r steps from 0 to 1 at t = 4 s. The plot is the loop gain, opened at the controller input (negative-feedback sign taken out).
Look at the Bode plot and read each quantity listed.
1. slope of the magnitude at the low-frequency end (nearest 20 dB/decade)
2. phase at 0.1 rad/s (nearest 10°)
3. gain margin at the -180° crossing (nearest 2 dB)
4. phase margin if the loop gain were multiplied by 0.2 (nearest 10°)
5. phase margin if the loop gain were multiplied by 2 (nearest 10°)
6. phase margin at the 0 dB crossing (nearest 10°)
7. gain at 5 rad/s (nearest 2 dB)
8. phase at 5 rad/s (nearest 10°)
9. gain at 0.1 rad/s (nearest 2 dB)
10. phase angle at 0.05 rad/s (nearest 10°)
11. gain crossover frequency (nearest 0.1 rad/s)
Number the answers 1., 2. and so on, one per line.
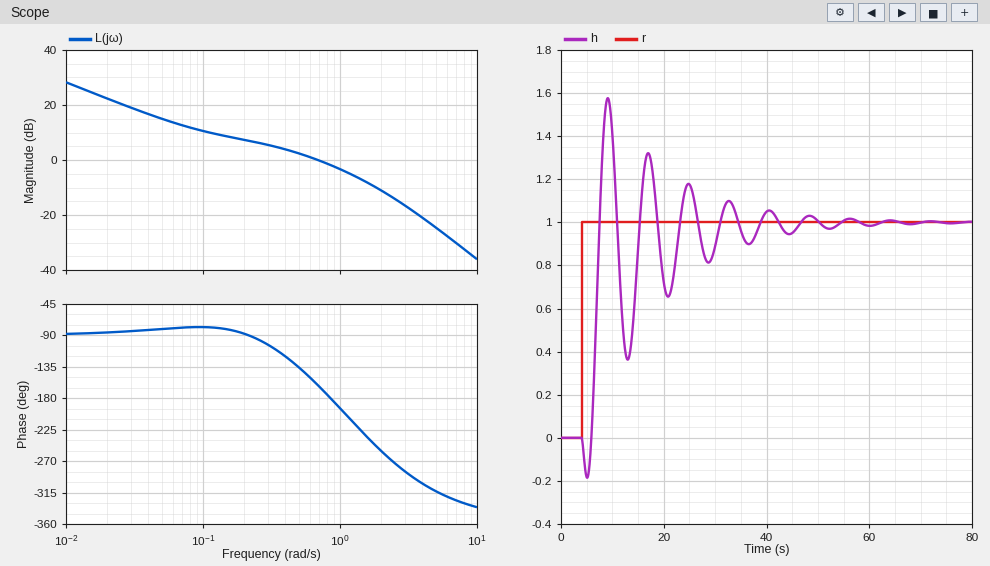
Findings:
1. -20 dB/decade
2. -80°
3. 2 dB
4. 100°
5. -40°
6. 20°
7. -24 dB
8. -310°
9. 10 dB
10. -80°
11. 0.7 rad/s
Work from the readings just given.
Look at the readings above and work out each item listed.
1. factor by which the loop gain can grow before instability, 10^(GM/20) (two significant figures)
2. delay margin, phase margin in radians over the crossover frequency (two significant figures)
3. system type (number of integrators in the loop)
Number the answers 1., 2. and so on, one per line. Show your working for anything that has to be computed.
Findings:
1. 10^(2 / 20) = 1.3
2. 20 × π / 180 / 0.7 = 0.50 s
3. 1
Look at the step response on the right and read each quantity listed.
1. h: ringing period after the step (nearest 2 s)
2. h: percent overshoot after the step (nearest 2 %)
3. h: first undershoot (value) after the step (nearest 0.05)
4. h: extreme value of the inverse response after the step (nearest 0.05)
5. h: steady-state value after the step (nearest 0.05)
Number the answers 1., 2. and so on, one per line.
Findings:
1. 8 s
2. 58 %
3. 0.35
4. -0.20
5. 1.00
